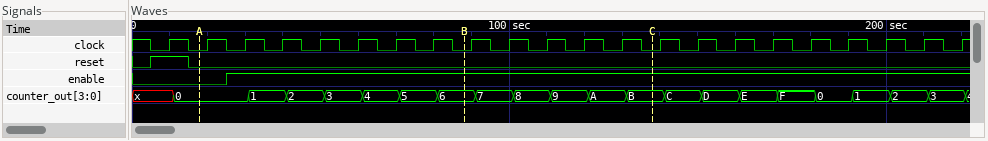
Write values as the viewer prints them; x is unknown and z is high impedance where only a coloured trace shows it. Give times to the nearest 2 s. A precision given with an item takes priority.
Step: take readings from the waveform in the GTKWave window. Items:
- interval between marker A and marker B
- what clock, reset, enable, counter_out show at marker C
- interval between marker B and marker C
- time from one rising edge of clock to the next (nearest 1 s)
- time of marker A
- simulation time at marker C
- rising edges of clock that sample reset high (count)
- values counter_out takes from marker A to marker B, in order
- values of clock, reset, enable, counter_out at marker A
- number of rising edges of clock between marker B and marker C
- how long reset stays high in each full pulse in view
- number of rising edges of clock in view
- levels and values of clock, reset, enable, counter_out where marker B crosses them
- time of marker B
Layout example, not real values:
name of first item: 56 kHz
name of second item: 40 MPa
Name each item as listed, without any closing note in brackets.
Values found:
interval between marker A and marker B: 70 s
what clock, reset, enable, counter_out show at marker C: clock=0, reset=0, enable=1, counter_out=B
interval between marker B and marker C: 50 s
time from one rising edge of clock to the next: 10 s
time of marker A: 18 s
simulation time at marker C: 138 s
rising edges of clock that sample reset high: 1
values counter_out takes from marker A to marker B, in order: 0, 1, 2, 3, 4, 5, 6
values of clock, reset, enable, counter_out at marker A: clock=0, reset=0, enable=0, counter_out=0
number of rising edges of clock between marker B and marker C: 5
how long reset stays high in each full pulse in view: 10 s
number of rising edges of clock in view: 22
levels and values of clock, reset, enable, counter_out where marker B crosses them: clock=0, reset=0, enable=1, counter_out=6
time of marker B: 88 s
